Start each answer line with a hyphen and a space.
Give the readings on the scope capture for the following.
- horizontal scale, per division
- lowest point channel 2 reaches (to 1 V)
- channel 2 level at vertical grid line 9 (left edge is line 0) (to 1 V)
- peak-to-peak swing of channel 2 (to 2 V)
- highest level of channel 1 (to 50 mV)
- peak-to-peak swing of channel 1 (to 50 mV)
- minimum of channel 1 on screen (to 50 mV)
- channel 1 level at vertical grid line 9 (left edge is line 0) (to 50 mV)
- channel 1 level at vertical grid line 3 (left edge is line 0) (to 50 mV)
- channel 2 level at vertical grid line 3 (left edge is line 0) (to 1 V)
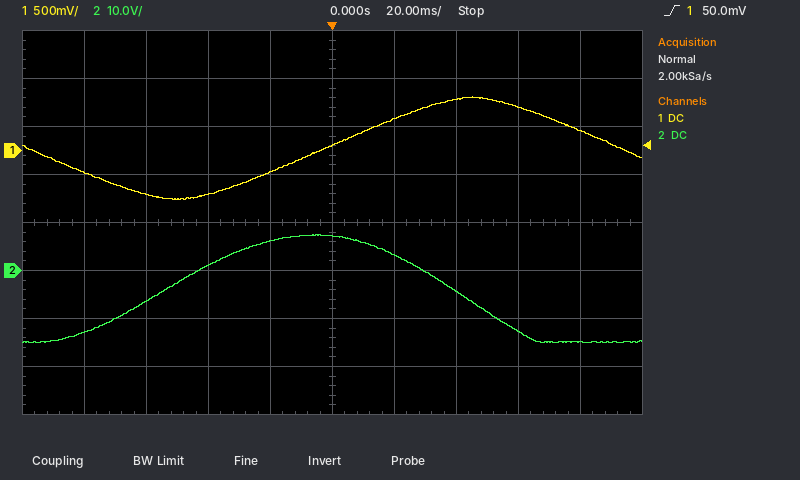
- 20 ms
- -15 V
- -15 V
- 22 V
- 550 mV
- 1.05 V
- -500 mV
- 200 mV
- -450 mV
- 1 V
